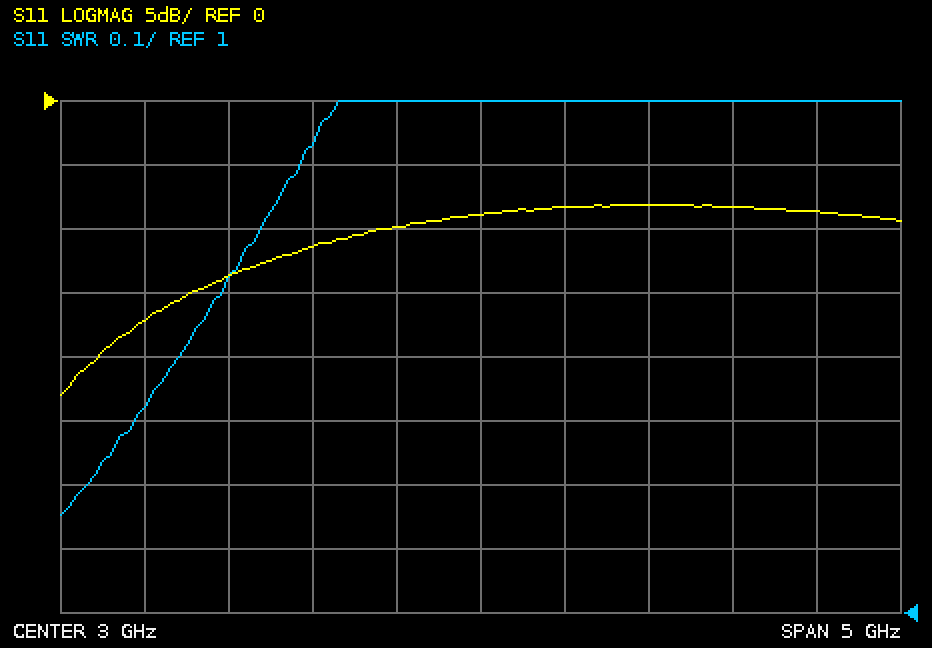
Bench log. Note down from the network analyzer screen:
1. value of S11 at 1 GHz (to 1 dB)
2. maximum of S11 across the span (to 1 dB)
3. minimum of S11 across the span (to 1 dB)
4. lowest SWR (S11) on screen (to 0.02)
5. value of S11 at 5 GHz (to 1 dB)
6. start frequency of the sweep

-17 dB
-8 dB
-23 dB
1.16
-9 dB
500 MHz
